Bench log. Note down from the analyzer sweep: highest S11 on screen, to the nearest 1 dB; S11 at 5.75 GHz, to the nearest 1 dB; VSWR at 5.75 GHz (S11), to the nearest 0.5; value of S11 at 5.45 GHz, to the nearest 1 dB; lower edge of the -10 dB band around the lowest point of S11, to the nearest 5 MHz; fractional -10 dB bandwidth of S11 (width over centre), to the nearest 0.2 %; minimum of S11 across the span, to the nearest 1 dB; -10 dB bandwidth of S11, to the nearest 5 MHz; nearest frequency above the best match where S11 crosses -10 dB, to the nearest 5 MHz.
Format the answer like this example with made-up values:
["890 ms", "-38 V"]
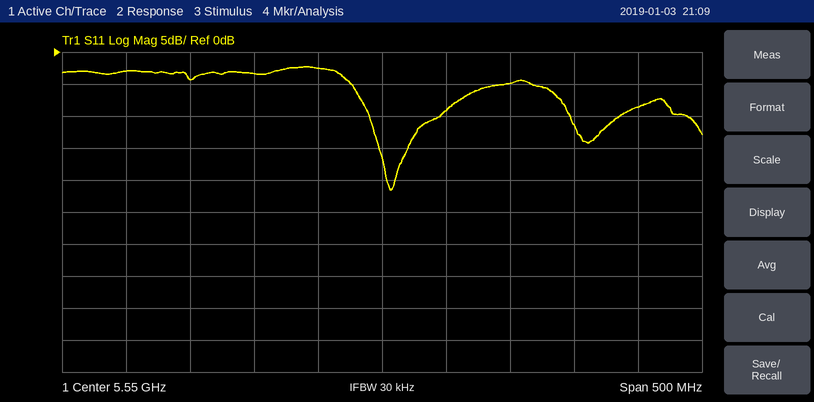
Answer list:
["-2 dB", "-9 dB", "2.0", "-3 dB", "5.540 GHz", "1.0 %", "-22 dB", "55 MHz", "5.595 GHz"]
